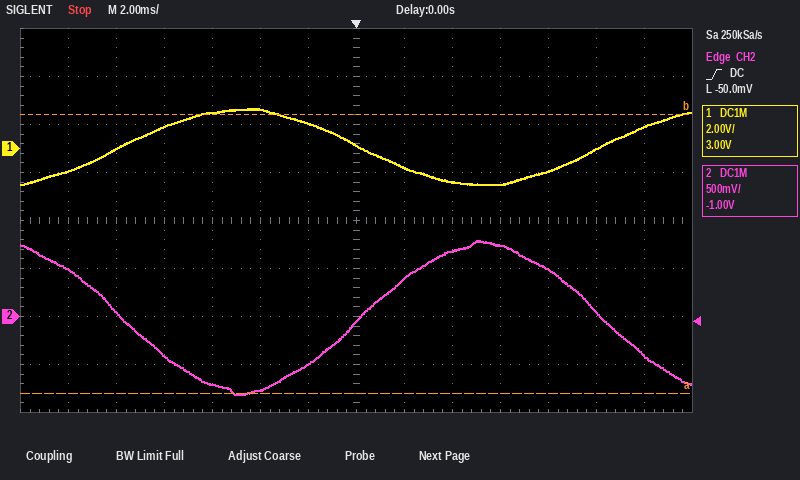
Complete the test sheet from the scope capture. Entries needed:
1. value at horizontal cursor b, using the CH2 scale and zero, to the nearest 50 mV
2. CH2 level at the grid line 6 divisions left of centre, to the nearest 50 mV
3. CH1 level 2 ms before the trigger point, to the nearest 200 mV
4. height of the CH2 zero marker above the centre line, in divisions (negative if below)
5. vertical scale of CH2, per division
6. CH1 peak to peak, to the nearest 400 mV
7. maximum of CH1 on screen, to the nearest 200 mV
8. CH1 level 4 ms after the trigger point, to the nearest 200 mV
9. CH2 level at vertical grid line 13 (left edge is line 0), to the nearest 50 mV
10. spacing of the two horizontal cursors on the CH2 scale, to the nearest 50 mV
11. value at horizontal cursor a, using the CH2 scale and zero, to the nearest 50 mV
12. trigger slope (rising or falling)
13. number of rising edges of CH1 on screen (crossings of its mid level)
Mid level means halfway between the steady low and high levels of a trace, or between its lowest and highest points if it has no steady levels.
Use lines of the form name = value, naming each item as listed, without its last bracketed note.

value at horizontal cursor b, using the CH2 scale and zero, to the nearest 50 mV = 2.10 V
CH2 level at the grid line 6 divisions left of centre, to the nearest 50 mV = 500 mV
CH1 level 2 ms before the trigger point, to the nearest 200 mV = 1.0 V
height of the CH2 zero marker above the centre line, in divisions = -2.0 div
vertical scale of CH2, per division = 500 mV
CH1 peak to peak, to the nearest 400 mV = 3.2 V
maximum of CH1 on screen, to the nearest 200 mV = 1.6 V
CH1 level 4 ms after the trigger point, to the nearest 200 mV = -1.4 V
CH2 level at vertical grid line 13 (left edge is line 0), to the nearest 50 mV = -400 mV
spacing of the two horizontal cursors on the CH2 scale, to the nearest 50 mV = 2.90 V
value at horizontal cursor a, using the CH2 scale and zero, to the nearest 50 mV = -800 mV
trigger slope = rising
number of rising edges of CH1 on screen = 2
